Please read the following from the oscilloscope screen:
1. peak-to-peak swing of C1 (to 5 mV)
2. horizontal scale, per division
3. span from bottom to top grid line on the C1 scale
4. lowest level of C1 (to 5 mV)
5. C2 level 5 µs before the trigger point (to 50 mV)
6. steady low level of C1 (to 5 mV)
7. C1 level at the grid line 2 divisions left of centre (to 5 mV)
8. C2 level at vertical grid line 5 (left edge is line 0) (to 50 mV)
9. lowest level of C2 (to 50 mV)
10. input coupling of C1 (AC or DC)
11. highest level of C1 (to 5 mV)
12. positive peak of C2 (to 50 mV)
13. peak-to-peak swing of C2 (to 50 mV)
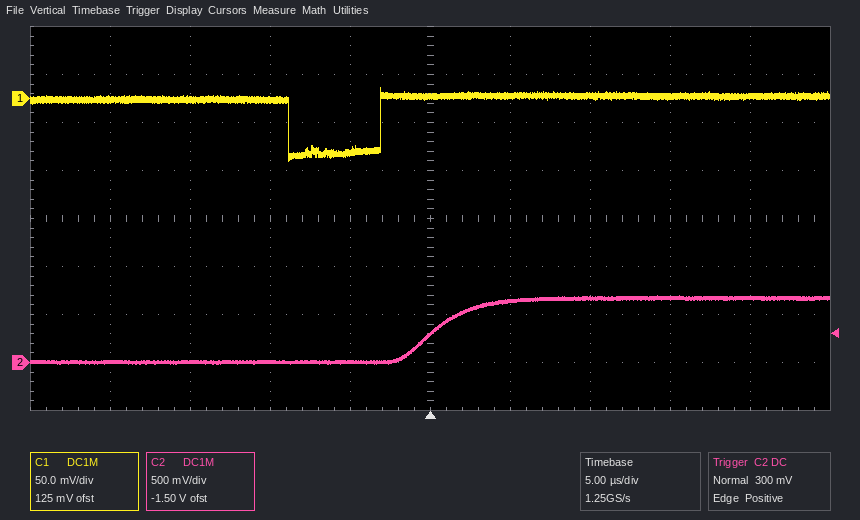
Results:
75 mV
5 µs
400 mV
-65 mV
0 mV
-55 mV
0 mV
300 mV
0 mV
DC
10 mV
700 mV
700 mV
